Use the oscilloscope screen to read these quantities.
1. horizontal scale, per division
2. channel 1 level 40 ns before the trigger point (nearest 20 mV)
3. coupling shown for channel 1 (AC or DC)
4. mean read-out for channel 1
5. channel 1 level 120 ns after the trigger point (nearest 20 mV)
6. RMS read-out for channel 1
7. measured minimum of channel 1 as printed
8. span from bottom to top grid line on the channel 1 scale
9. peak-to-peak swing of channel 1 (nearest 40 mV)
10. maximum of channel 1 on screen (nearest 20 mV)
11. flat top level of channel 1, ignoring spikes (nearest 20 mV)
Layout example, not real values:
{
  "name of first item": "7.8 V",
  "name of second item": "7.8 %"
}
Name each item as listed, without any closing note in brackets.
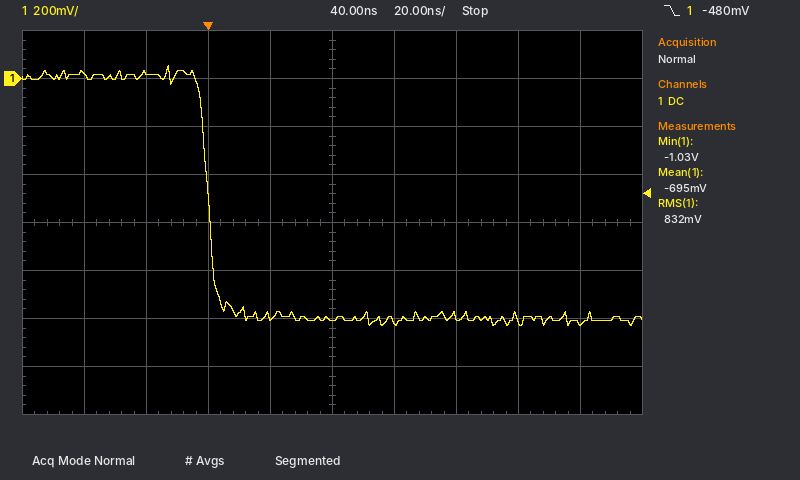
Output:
{
  "horizontal scale, per division": "20 ns",
  "channel 1 level 40 ns before the trigger point": "20 mV",
  "coupling shown for channel 1": "DC",
  "mean read-out for channel 1": "-695 mV",
  "channel 1 level 120 ns after the trigger point": "-1.02 V",
  "RMS read-out for channel 1": "832 mV",
  "measured minimum of channel 1 as printed": "-1.03 V",
  "span from bottom to top grid line on the channel 1 scale": "1.6 V",
  "peak-to-peak swing of channel 1": "1.08 V",
  "maximum of channel 1 on screen": "60 mV",
  "flat top level of channel 1, ignoring spikes": "20 mV"
}
